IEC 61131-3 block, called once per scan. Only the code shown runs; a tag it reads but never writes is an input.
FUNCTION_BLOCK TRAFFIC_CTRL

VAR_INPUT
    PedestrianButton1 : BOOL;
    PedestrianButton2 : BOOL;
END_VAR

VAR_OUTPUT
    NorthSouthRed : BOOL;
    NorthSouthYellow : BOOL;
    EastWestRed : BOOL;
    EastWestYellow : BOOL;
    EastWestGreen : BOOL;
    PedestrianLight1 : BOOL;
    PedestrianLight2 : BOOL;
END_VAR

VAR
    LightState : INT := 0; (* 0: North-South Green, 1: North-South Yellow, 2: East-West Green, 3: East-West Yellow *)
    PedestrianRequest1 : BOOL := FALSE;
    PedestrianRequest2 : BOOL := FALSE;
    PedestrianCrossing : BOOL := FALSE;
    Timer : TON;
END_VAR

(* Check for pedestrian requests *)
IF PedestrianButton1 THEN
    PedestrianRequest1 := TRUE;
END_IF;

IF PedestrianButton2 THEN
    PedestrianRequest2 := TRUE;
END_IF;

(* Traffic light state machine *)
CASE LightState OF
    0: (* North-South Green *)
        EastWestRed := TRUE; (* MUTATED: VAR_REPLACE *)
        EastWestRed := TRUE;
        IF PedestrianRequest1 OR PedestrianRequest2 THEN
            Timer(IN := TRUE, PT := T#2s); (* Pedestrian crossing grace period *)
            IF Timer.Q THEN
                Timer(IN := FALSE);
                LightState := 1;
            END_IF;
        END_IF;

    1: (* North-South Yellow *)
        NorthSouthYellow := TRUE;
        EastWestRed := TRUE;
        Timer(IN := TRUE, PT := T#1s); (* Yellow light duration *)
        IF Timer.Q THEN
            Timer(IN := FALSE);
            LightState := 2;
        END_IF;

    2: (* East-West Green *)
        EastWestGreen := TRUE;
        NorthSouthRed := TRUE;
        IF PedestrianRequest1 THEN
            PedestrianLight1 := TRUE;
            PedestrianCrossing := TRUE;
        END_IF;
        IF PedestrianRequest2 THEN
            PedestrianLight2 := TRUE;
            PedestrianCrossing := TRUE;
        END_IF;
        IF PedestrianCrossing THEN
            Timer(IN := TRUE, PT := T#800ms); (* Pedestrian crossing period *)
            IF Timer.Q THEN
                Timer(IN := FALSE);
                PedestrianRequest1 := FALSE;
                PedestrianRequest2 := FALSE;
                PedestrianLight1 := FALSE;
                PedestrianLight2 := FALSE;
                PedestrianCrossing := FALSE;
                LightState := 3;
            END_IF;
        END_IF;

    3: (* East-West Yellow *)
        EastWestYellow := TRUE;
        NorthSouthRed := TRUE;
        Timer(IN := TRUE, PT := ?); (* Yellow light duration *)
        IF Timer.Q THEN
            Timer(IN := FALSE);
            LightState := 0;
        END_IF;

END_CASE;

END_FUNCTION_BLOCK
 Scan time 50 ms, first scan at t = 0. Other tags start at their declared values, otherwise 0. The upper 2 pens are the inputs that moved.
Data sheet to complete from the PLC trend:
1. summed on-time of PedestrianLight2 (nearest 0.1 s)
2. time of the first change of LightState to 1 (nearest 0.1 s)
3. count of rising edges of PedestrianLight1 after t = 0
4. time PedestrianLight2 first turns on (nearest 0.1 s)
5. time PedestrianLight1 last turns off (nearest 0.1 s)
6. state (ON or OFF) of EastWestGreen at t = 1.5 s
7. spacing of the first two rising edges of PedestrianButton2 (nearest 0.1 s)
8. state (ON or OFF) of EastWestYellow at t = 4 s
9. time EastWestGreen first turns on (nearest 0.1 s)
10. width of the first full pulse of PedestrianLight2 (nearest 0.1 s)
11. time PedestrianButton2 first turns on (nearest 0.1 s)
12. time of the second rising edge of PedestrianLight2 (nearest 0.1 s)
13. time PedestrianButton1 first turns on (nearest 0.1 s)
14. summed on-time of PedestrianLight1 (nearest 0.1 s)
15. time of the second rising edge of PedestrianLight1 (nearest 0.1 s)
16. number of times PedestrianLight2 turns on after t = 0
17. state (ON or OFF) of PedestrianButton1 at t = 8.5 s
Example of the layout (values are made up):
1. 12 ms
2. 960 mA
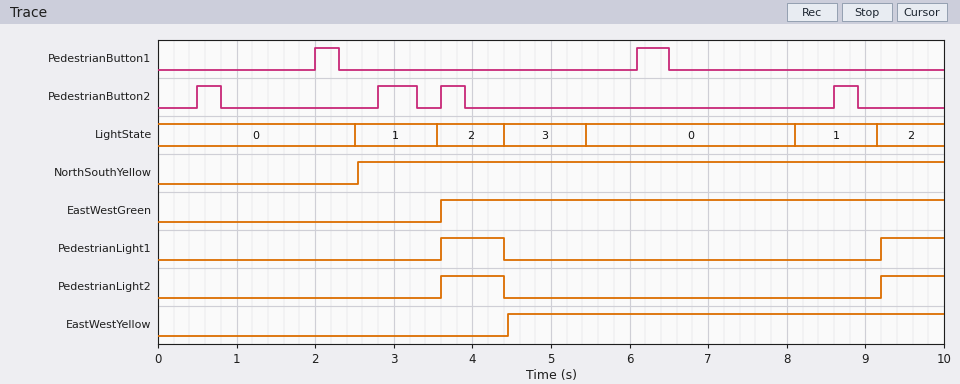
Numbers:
1. 1.6 s
2. 2.5 s
3. 2
4. 3.6 s
5. 4.4 s
6. OFF
7. 2.3 s
8. OFF
9. 3.6 s
10. 0.8 s
11. 0.5 s
12. 9.2 s
13. 2.0 s
14. 1.6 s
15. 9.2 s
16. 2
17. OFF
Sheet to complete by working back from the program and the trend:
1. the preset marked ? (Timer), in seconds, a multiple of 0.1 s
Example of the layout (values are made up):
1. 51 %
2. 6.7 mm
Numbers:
1. 1.0 s
